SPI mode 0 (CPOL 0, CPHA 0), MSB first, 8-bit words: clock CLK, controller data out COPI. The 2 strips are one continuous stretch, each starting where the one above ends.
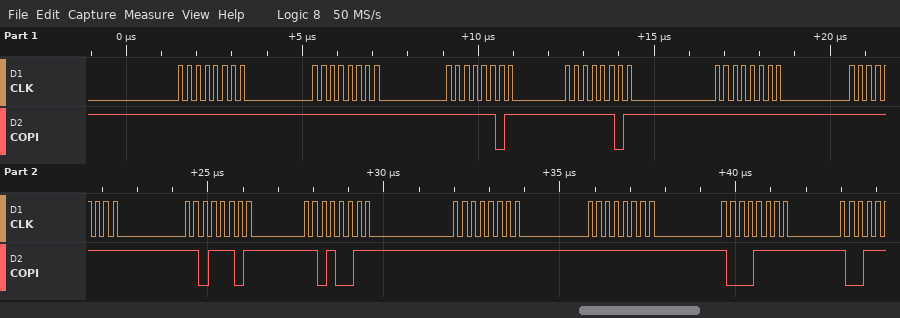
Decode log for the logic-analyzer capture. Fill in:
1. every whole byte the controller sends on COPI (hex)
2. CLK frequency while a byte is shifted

FF FF FD FD FF FF DD D3 FF FF 8F
4 MHz
